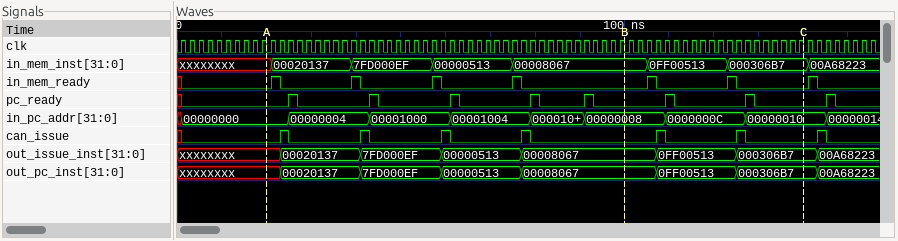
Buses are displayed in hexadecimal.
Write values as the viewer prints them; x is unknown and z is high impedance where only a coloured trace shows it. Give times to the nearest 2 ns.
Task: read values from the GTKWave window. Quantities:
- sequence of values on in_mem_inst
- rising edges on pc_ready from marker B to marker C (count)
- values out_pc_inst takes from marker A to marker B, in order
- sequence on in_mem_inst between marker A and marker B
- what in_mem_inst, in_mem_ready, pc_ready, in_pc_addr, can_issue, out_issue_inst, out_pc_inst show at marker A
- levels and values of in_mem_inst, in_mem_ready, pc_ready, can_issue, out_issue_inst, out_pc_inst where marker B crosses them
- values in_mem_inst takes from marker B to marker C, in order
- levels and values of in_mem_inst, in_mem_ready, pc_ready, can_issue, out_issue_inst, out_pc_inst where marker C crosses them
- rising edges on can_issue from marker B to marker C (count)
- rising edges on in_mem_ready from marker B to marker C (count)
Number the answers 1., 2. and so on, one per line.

1. xxxxxxxx, 00020137, 7FD000EF, 00000513, 00008067, 0FF00513, 000306B7, 00A68223
2. 2
3. xxxxxxxx, 00020137, 7FD000EF, 00000513, 00008067
4. xxxxxxxx, 00020137, 7FD000EF, 00000513, 00008067
5. in_mem_inst=xxxxxxxx, in_mem_ready=0, pc_ready=0, in_pc_addr=00000000, can_issue=0, out_issue_inst=xxxxxxxx, out_pc_inst=xxxxxxxx
6. in_mem_inst=00008067, in_mem_ready=0, pc_ready=0, can_issue=0, out_issue_inst=00008067, out_pc_inst=00008067
7. 00008067, 0FF00513, 000306B7
8. in_mem_inst=000306B7, in_mem_ready=0, pc_ready=0, can_issue=0, out_issue_inst=000306B7, out_pc_inst=000306B7
9. 2
10. 2
